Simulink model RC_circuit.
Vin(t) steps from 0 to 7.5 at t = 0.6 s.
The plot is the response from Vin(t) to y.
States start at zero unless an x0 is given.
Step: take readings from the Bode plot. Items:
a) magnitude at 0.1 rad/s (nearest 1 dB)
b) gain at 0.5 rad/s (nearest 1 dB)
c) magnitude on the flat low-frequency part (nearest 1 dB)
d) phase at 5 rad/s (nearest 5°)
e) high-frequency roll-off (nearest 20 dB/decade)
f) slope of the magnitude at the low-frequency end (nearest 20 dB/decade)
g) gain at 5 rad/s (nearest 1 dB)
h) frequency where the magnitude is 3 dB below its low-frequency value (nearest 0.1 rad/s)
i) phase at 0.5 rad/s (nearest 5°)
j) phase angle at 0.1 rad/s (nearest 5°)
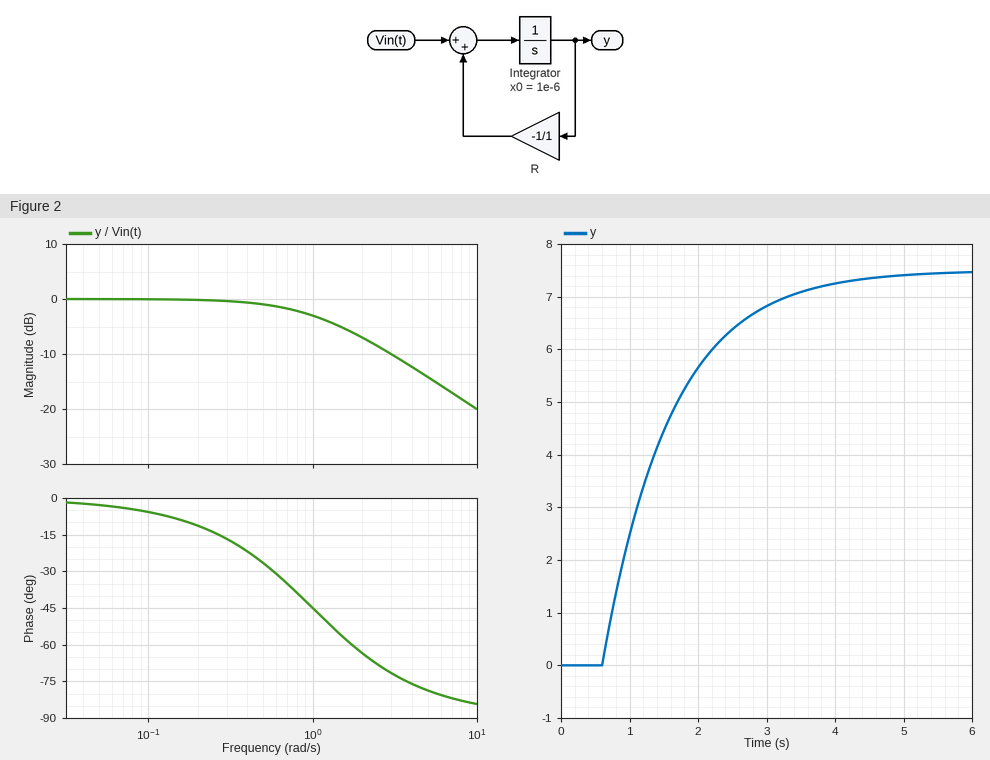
0 dB
-1 dB
0 dB
-80°
-20 dB/decade
0 dB/decade
-14 dB
1.0 rad/s
-25°
-5°
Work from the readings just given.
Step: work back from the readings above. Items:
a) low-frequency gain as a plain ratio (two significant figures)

1.0
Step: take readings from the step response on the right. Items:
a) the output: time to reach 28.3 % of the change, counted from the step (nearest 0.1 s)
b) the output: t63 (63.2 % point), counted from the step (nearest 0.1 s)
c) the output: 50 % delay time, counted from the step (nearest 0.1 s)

0.3 s
1.0 s
0.7 s
